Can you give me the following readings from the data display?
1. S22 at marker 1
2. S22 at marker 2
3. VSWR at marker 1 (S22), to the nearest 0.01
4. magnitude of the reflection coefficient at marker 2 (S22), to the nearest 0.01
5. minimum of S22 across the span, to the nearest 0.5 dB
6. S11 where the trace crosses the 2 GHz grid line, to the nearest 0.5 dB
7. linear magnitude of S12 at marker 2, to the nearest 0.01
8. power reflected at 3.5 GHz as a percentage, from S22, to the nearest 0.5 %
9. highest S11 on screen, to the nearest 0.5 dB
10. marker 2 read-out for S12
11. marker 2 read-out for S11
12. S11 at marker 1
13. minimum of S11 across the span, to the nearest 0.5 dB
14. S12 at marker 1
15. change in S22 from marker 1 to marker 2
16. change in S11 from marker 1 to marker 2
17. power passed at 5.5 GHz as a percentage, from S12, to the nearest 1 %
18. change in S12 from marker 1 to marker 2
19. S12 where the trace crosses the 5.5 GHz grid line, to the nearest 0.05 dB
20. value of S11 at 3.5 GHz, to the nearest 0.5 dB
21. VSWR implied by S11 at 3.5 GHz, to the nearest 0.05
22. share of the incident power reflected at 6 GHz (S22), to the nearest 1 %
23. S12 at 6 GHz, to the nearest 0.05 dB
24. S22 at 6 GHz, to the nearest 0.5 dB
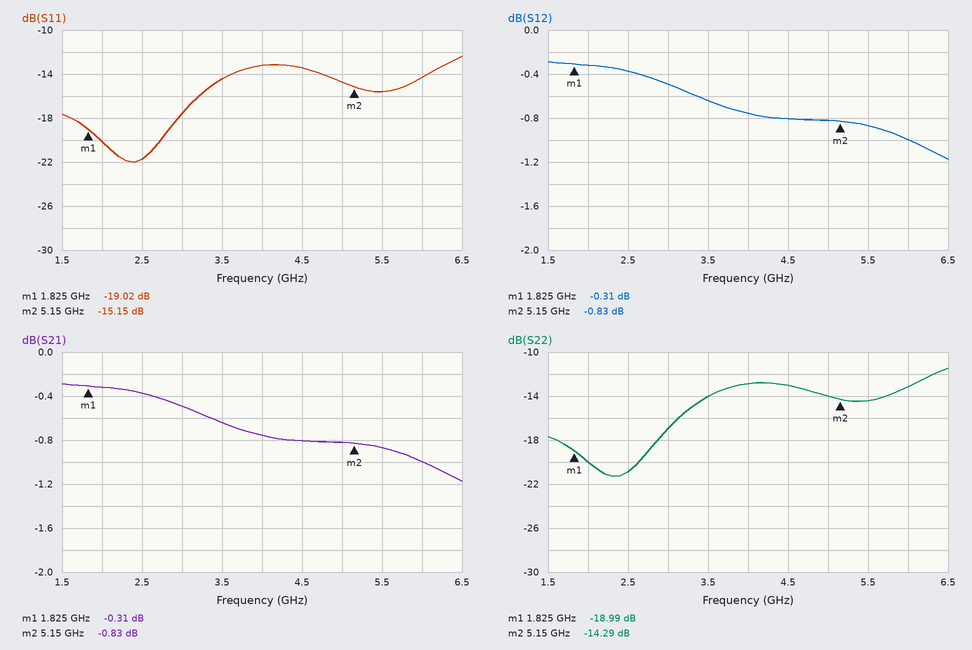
-18.99 dB
-14.29 dB
1.25
0.19
-21.5 dB
-20.0 dB
0.91
4.0 %
-12.5 dB
-0.83 dB
-15.15 dB
-19.02 dB
-22.0 dB
-0.31 dB
4.70 dB
3.87 dB
82 %
-0.52 dB
-0.85 dB
-14.5 dB
1.45
5 %
-1.00 dB
-13.0 dB
